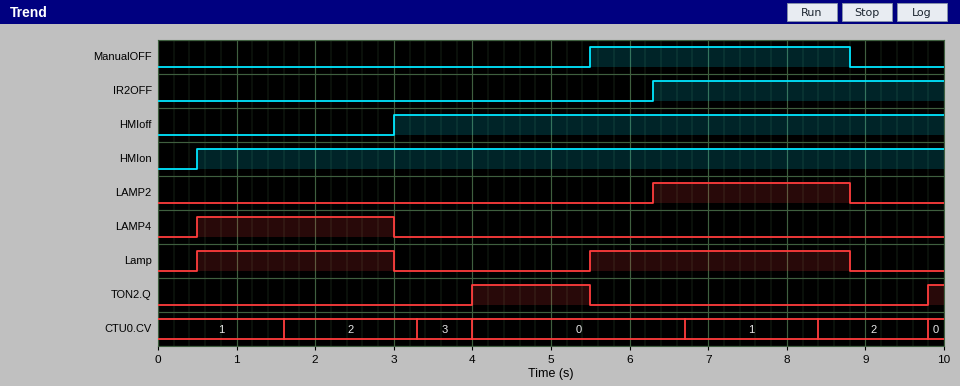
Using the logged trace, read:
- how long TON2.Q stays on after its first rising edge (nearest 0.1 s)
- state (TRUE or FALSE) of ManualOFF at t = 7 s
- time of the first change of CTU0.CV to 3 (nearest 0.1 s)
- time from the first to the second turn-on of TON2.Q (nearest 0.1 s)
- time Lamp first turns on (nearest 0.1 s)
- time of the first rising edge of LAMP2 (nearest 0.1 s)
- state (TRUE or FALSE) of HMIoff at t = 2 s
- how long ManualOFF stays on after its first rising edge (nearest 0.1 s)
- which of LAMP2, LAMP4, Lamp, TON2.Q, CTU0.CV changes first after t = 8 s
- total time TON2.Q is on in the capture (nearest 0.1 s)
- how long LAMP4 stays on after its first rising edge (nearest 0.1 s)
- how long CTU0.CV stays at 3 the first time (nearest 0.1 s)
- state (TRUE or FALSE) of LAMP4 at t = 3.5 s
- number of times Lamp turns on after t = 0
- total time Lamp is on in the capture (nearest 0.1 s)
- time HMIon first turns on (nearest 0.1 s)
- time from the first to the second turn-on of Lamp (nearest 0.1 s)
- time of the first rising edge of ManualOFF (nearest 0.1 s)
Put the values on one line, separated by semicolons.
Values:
1.5 s; TRUE; 3.3 s; 5.8 s; 0.5 s; 6.3 s; FALSE; 3.3 s; CTU0.CV; 1.7 s; 2.5 s; 0.7 s; FALSE; 2; 5.8 s; 0.5 s; 5.0 s; 5.5 s
